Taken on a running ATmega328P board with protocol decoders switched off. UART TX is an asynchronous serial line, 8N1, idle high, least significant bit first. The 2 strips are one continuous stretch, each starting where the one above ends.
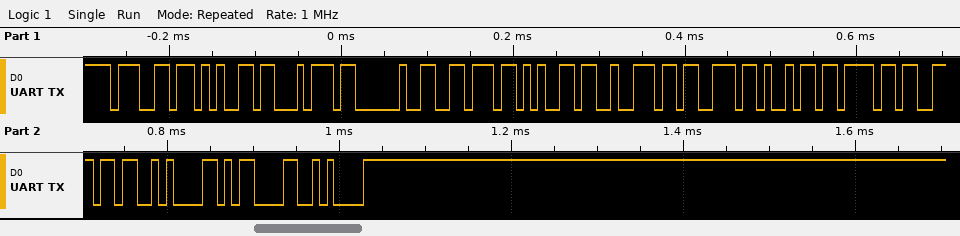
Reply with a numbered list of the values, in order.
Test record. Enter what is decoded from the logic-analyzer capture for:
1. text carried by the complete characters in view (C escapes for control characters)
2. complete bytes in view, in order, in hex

1. "get version\n\r\n"
2. 0x67 0x65 0x74 0x20 0x76 0x65 0x72 0x73 0x69 0x6F 0x6E 0x0A 0x0D 0x0A
